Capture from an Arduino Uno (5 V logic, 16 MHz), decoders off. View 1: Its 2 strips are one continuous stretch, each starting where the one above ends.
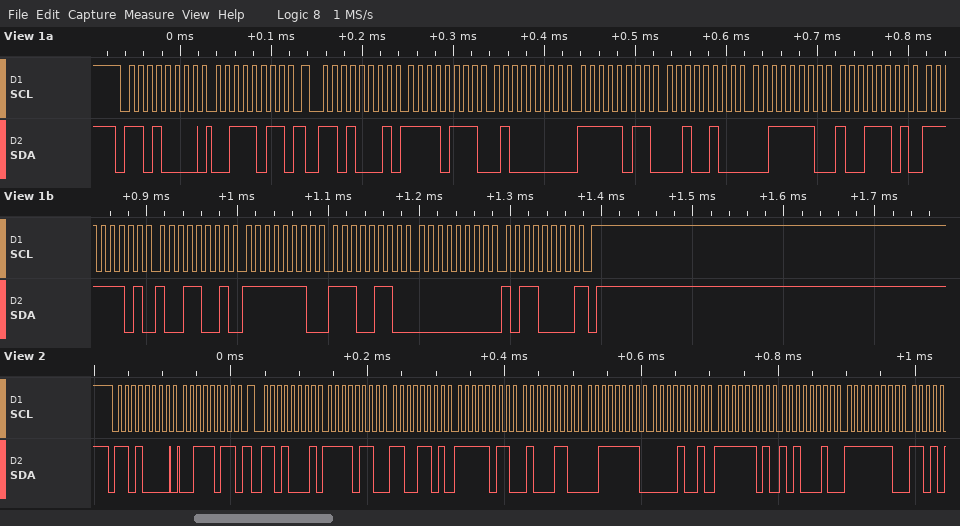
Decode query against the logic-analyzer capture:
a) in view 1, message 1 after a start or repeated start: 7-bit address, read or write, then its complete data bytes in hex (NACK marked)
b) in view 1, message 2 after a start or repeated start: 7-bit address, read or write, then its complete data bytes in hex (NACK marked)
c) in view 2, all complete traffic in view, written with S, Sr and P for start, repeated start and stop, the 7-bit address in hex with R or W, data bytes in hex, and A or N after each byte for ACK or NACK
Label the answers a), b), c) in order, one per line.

a) 0x68 write: 3B
b) 0x68 read: F7 40 FB 24 3E 9D FD 99 FE E6 00 B0 NACK
c) S 68W A 3B A Sr 68R A F6 A CD A FB A 46 A 3F A 09 A FD A A2 A FE A
